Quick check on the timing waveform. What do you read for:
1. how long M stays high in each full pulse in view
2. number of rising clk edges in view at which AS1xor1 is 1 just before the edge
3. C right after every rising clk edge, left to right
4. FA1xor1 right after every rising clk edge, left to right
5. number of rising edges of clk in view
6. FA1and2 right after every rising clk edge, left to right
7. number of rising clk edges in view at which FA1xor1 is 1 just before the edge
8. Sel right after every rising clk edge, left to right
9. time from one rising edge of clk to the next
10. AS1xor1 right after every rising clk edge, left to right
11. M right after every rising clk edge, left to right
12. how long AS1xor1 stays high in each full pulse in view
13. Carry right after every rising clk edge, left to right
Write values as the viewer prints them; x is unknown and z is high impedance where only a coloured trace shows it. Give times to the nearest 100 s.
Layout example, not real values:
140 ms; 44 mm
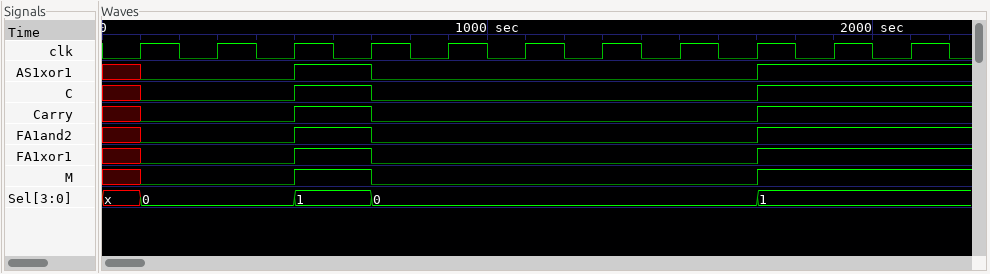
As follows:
200 s; 3; 0 0 1 0 0 0 0 0 1 1 1; 0 0 1 0 0 0 0 0 1 1 1; 11; 0 0 1 0 0 0 0 0 1 1 1; 3; 0, 0, 1, 0, 0, 0, 0, 0, 1, 1, 1; 200 s; 0 0 1 0 0 0 0 0 1 1 1; 0 0 1 0 0 0 0 0 1 1 1; 200 s; 0 0 1 0 0 0 0 0 1 1 1
